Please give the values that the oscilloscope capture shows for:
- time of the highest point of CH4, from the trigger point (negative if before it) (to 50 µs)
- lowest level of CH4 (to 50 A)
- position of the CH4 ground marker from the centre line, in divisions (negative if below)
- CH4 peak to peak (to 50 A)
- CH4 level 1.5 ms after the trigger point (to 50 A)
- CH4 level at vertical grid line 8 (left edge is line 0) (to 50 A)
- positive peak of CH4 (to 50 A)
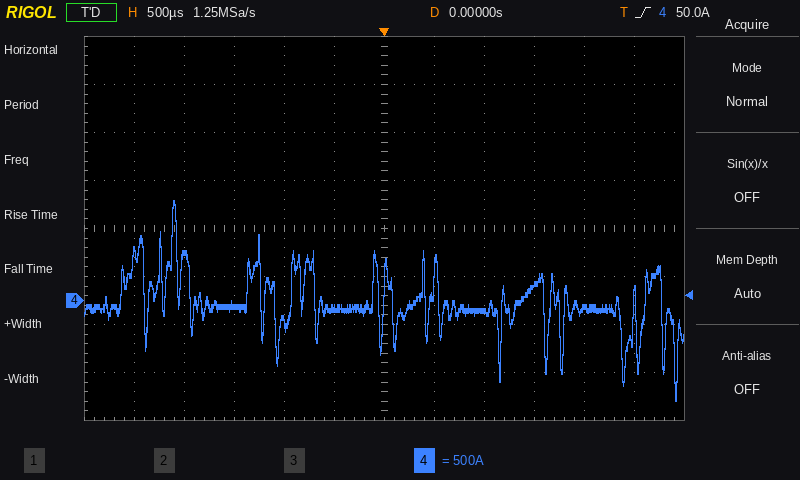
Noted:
-2.10 ms
-1.05 kA
-1.5 div
2.10 kA
150 A
-100 A
1.05 kA
